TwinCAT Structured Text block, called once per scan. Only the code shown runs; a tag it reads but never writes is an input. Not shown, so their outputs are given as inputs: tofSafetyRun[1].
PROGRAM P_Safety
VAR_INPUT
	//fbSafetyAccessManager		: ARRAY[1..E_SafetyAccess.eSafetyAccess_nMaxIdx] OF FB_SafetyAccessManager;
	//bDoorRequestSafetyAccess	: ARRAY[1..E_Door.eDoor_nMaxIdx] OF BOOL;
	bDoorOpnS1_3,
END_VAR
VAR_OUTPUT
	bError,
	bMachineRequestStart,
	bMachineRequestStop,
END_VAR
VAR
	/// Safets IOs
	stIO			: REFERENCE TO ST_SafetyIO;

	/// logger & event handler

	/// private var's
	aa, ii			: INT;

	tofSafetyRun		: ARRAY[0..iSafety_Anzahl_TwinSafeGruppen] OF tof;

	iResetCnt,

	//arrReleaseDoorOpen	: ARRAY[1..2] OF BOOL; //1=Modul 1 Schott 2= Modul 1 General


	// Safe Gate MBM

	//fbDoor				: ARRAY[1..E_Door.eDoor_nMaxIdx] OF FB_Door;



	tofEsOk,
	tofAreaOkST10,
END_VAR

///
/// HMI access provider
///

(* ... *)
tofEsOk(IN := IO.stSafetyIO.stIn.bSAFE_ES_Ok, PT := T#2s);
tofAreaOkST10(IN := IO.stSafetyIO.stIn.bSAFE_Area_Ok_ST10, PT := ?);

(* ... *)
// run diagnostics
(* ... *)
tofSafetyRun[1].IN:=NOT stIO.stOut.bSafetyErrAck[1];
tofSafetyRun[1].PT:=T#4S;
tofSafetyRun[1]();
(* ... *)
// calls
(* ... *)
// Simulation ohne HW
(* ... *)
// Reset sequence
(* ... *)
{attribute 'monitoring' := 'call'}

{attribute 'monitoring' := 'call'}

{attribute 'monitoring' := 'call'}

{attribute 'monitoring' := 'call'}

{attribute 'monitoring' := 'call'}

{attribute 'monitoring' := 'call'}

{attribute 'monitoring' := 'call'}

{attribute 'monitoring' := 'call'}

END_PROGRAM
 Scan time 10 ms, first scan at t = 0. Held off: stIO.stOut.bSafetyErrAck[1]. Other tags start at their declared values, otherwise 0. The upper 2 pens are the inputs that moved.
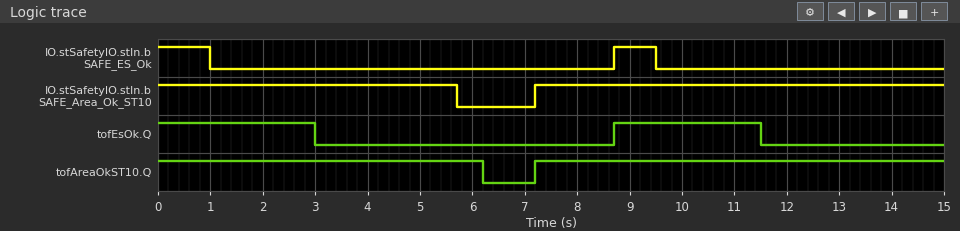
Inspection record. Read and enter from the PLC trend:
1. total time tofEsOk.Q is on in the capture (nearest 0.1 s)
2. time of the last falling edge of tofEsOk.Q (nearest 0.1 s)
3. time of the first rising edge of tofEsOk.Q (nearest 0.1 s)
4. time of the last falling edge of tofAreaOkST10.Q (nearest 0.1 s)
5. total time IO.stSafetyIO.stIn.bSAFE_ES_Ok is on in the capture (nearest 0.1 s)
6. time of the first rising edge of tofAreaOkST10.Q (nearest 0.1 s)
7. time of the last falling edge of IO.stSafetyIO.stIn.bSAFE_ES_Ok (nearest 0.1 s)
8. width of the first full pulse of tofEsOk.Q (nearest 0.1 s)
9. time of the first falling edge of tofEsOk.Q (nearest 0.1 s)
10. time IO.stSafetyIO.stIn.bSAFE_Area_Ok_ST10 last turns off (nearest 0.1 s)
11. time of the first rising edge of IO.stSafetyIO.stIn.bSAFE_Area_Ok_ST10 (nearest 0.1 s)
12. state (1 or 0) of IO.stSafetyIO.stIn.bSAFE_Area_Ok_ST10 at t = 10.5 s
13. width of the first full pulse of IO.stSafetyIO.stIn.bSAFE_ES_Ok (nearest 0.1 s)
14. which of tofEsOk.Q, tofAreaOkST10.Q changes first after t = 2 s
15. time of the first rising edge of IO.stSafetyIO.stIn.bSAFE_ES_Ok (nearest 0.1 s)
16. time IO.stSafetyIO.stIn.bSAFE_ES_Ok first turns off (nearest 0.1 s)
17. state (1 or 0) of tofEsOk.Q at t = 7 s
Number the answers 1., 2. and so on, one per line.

1. 5.8 s
2. 11.5 s
3. 8.7 s
4. 6.2 s
5. 1.8 s
6. 7.2 s
7. 9.5 s
8. 2.8 s
9. 3.0 s
10. 5.7 s
11. 7.2 s
12. 1
13. 0.8 s
14. tofEsOk.Q
15. 8.7 s
16. 1.0 s
17. 0
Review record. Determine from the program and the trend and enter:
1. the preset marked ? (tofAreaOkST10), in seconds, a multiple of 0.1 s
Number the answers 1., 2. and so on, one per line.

1. 0.5 s
